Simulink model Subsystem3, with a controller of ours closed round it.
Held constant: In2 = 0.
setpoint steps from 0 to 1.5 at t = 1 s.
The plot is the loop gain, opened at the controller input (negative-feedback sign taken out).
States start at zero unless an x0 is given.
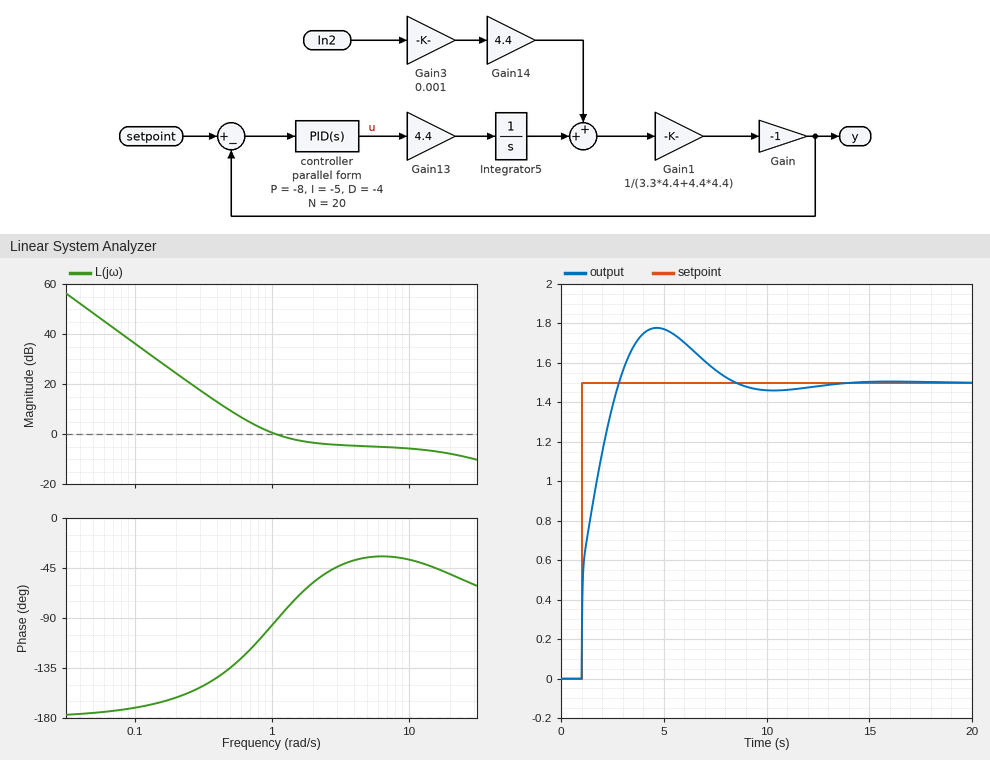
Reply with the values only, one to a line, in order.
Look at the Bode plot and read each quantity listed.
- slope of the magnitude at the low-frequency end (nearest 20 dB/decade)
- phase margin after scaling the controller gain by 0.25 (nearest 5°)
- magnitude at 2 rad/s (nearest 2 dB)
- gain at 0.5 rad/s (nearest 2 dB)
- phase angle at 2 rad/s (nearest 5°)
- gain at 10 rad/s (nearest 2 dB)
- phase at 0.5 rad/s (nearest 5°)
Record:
-40 dB/decade
40°
-4 dB
10 dB
-60°
-6 dB
-135°
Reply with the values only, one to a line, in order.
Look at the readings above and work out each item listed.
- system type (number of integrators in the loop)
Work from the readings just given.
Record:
2
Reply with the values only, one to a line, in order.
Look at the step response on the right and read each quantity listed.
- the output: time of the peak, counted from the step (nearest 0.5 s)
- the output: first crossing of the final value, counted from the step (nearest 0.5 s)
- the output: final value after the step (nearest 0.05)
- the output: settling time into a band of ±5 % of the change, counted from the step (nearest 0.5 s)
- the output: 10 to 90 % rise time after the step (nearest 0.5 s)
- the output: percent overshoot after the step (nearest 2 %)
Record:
3.5 s
2.0 s
1.50
6.5 s
1.5 s
18 %
